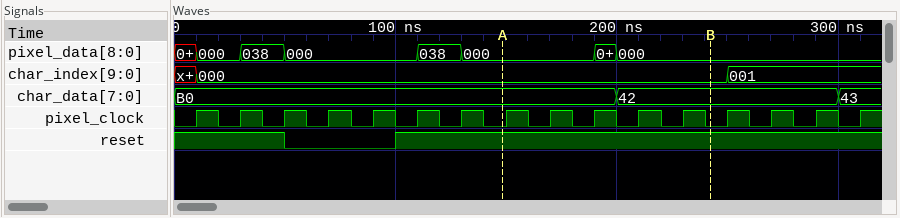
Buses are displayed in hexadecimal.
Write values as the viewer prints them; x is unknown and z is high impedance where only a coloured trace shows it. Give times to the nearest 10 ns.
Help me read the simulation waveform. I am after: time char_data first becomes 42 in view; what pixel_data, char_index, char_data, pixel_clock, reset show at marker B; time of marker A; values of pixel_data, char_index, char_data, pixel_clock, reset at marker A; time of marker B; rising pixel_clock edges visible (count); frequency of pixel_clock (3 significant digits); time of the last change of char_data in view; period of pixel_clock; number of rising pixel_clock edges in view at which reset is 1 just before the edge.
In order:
200 ns
pixel_data=000, char_index=000, char_data=42, pixel_clock=0, reset=1
150 ns
pixel_data=000, char_index=000, char_data=B0, pixel_clock=0, reset=1
240 ns
16
50.0 MHz
300 ns
20 ns
14
